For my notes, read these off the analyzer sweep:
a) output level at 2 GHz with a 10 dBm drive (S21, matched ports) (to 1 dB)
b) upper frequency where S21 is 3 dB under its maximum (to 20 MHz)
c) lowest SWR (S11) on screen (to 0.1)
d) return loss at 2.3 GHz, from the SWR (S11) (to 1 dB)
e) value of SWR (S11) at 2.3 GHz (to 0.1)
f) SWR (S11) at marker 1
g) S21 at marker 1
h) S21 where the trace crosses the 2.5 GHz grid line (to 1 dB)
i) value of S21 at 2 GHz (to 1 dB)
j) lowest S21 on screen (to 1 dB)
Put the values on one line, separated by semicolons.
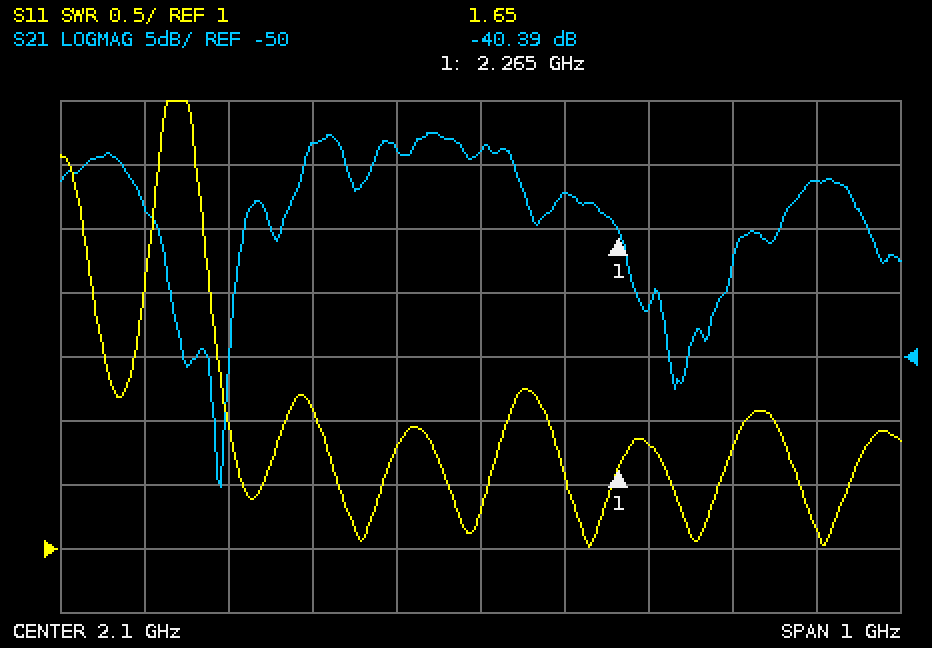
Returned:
-24 dBm; 2.14 GHz; 1.0; 11 dB; 1.8; 1.65; -40.39 dB; -36 dB; -34 dB; -60 dB
